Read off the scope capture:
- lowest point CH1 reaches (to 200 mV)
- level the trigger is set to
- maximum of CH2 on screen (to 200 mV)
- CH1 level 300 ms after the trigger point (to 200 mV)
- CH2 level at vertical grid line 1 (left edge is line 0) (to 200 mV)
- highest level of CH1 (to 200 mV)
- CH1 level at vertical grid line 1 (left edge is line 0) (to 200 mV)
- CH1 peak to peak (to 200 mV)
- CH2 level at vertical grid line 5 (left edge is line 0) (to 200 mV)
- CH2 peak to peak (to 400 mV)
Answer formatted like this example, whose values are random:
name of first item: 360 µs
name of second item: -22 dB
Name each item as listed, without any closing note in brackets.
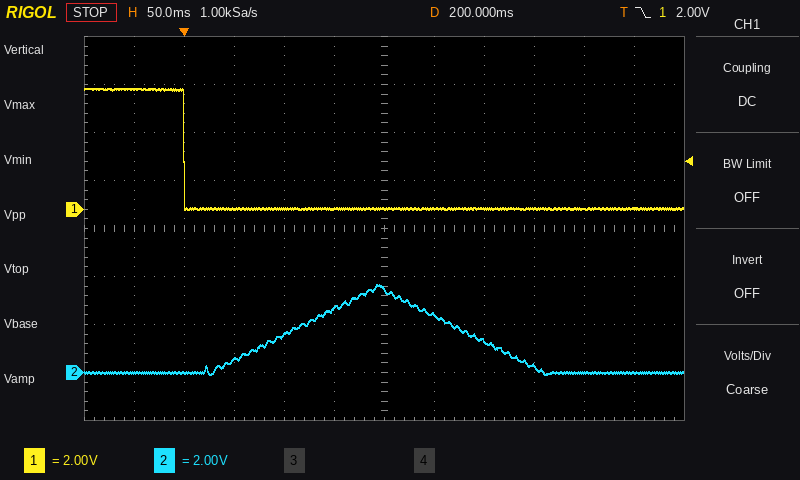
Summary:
lowest point CH1 reaches: 0.0 V
level the trigger is set to: 2.00 V
maximum of CH2 on screen: 3.6 V
CH1 level 300 ms after the trigger point: 0.0 V
CH2 level at vertical grid line 1 (left edge is line 0): 0.0 V
highest level of CH1: 5.0 V
CH1 level at vertical grid line 1 (left edge is line 0): 5.0 V
CH1 peak to peak: 5.0 V
CH2 level at vertical grid line 5 (left edge is line 0): 2.6 V
CH2 peak to peak: 3.6 V
